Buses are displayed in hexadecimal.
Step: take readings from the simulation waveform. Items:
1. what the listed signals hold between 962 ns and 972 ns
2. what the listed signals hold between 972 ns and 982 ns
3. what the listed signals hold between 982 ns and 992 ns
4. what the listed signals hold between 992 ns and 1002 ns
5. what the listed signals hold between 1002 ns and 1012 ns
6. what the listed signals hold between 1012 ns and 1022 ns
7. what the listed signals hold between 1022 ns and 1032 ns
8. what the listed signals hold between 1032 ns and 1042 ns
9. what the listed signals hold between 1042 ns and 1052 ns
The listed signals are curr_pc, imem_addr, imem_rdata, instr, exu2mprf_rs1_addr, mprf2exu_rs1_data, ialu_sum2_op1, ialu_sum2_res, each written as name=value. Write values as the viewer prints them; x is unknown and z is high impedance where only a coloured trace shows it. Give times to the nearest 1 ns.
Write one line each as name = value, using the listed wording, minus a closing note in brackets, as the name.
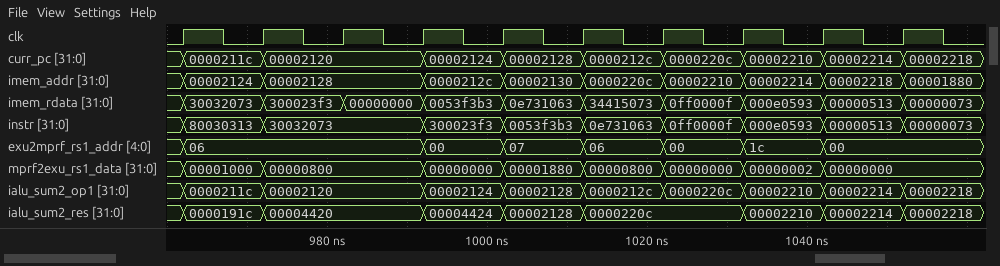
what the listed signals hold between 962 ns and 972 ns = curr_pc=0000211c, imem_addr=00002124, imem_rdata=30032073, instr=80030313, exu2mprf_rs1_addr=06, mprf2exu_rs1_data=00001000, ialu_sum2_op1=0000211c, ialu_sum2_res=0000191c
what the listed signals hold between 972 ns and 982 ns = curr_pc=00002120, imem_addr=00002128, imem_rdata=300023f3, instr=30032073, exu2mprf_rs1_addr=06, mprf2exu_rs1_data=00000800, ialu_sum2_op1=00002120, ialu_sum2_res=00004420
what the listed signals hold between 982 ns and 992 ns = curr_pc=00002120, imem_addr=00002128, imem_rdata=00000000, instr=30032073, exu2mprf_rs1_addr=06, mprf2exu_rs1_data=00000800, ialu_sum2_op1=00002120, ialu_sum2_res=00004420
what the listed signals hold between 992 ns and 1002 ns = curr_pc=00002124, imem_addr=0000212c, imem_rdata=0053f3b3, instr=300023f3, exu2mprf_rs1_addr=00, mprf2exu_rs1_data=00000000, ialu_sum2_op1=00002124, ialu_sum2_res=00004424
what the listed signals hold between 1002 ns and 1012 ns = curr_pc=00002128, imem_addr=00002130, imem_rdata=0e731063, instr=0053f3b3, exu2mprf_rs1_addr=07, mprf2exu_rs1_data=00001880, ialu_sum2_op1=00002128, ialu_sum2_res=00002128
what the listed signals hold between 1012 ns and 1022 ns = curr_pc=0000212c, imem_addr=0000220c, imem_rdata=34415073, instr=0e731063, exu2mprf_rs1_addr=06, mprf2exu_rs1_data=00000800, ialu_sum2_op1=0000212c, ialu_sum2_res=0000220c
what the listed signals hold between 1022 ns and 1032 ns = curr_pc=0000220c, imem_addr=00002210, imem_rdata=0ff0000f, instr=0ff0000f, exu2mprf_rs1_addr=00, mprf2exu_rs1_data=00000000, ialu_sum2_op1=0000220c, ialu_sum2_res=0000220c
what the listed signals hold between 1032 ns and 1042 ns = curr_pc=00002210, imem_addr=00002214, imem_rdata=000e0593, instr=000e0593, exu2mprf_rs1_addr=1c, mprf2exu_rs1_data=00000002, ialu_sum2_op1=00002210, ialu_sum2_res=00002210
what the listed signals hold between 1042 ns and 1052 ns = curr_pc=00002214, imem_addr=00002218, imem_rdata=00000513, instr=00000513, exu2mprf_rs1_addr=00, mprf2exu_rs1_data=00000000, ialu_sum2_op1=00002214, ialu_sum2_res=00002214
